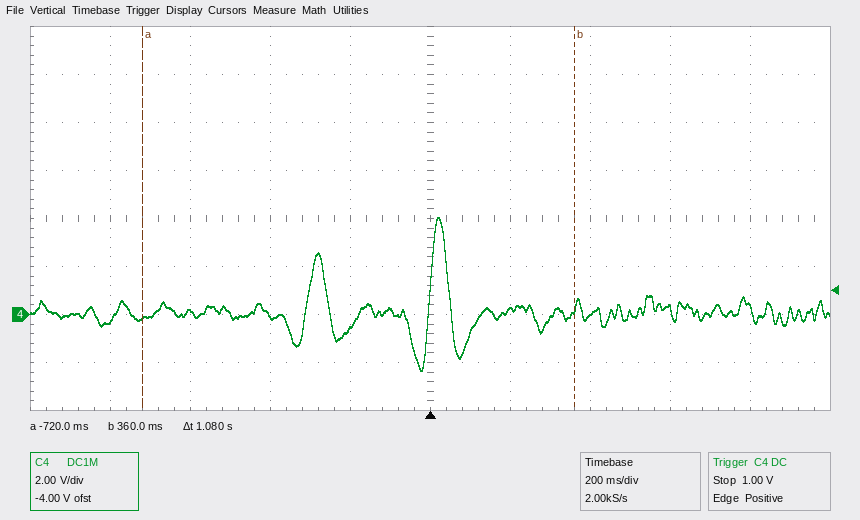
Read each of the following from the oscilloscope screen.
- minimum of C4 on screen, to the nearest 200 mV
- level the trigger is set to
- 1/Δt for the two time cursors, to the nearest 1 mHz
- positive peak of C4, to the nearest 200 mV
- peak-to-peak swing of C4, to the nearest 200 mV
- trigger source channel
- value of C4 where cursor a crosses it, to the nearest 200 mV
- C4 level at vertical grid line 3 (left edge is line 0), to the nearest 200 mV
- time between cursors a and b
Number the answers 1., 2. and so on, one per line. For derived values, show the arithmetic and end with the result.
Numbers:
1. -2.4 V
2. 1.00 V
3. 1 / 1.08 s ≈ 926 mHz
4. 4.0 V
5. 4.0 V − (-2.4 V) = 6.4 V
6. C4
7. -200 mV
8. 0.0 V
9. 1.08 s
